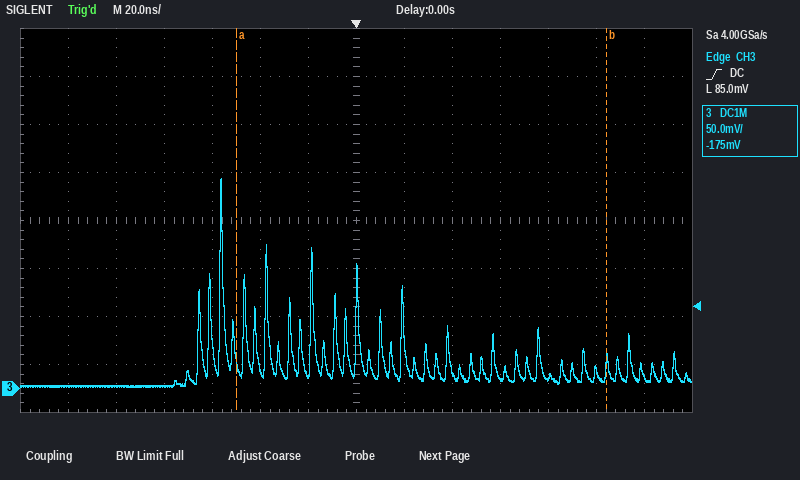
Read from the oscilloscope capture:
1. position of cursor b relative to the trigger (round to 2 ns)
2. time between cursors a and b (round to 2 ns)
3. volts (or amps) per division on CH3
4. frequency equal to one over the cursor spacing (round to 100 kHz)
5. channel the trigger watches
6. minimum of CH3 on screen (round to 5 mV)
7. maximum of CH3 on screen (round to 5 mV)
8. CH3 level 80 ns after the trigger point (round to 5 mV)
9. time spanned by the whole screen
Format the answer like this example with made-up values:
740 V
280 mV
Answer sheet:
+104 ns
154 ns
50 mV
6.5 MHz
CH3
0 mV
220 mV
10 mV
280 ns
